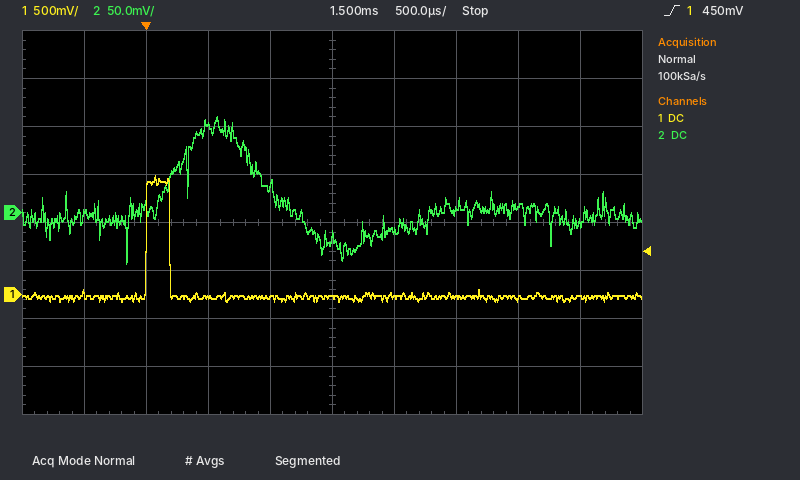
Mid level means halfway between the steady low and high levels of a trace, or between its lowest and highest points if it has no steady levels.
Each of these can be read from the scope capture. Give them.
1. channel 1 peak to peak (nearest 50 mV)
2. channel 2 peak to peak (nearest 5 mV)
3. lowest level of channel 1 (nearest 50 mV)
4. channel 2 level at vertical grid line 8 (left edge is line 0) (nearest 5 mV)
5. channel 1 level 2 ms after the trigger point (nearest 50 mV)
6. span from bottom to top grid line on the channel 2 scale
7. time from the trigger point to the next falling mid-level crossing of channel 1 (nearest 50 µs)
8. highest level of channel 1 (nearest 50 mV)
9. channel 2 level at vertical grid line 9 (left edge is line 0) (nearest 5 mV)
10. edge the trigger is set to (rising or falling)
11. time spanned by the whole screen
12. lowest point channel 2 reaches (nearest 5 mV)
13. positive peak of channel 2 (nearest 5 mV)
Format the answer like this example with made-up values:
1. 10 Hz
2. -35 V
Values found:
1. 1.30 V
2. 155 mV
3. -50 mV
4. 5 mV
5. 0 mV
6. 400 mV
7. 200 µs
8. 1.25 V
9. -10 mV
10. rising
11. 5 ms
12. -55 mV
13. 100 mV
